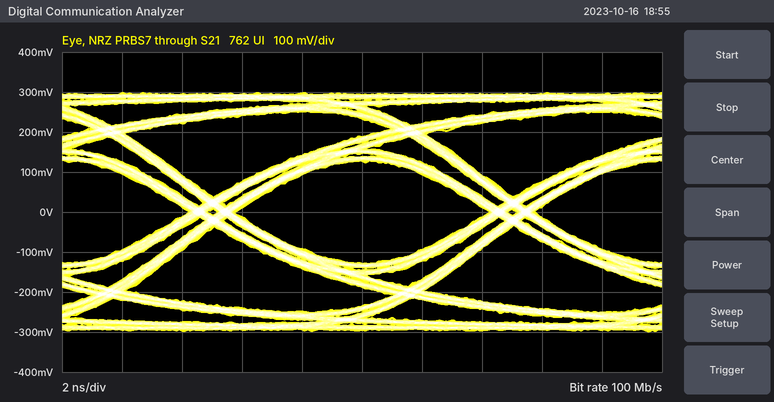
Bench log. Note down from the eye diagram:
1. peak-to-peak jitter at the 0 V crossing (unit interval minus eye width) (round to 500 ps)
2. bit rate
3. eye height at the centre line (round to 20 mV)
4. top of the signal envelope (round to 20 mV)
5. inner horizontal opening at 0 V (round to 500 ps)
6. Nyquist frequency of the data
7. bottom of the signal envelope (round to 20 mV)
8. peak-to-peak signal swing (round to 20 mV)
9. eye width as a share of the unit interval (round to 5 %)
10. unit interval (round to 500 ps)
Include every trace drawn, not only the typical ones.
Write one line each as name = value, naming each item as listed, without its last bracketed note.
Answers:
peak-to-peak jitter at the 0 V crossing (unit interval minus eye width) = 1.5 ns
bit rate = 100 Mb/s
eye height at the centre line = 260 mV
top of the signal envelope = 300 mV
inner horizontal opening at 0 V = 8.5 ns
Nyquist frequency of the data = 50 MHz
bottom of the signal envelope = -300 mV
peak-to-peak signal swing = 600 mV
eye width as a share of the unit interval = 85 %
unit interval = 10.0 ns
